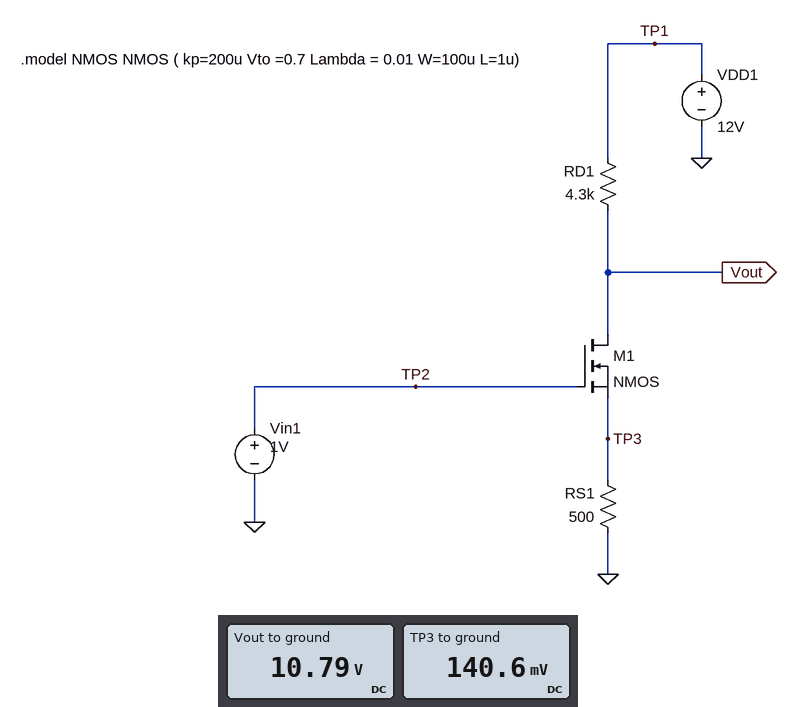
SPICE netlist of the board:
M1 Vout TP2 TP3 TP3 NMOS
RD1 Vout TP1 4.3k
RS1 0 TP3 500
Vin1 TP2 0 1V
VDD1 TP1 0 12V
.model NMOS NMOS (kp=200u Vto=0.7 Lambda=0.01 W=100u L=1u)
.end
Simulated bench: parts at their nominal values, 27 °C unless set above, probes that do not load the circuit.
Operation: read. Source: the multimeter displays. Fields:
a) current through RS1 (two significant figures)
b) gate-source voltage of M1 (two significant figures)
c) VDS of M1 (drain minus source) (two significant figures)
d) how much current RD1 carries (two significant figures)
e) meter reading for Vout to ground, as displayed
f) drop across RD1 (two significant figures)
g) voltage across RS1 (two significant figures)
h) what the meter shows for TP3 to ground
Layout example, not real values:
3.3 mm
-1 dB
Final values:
280 µA
860 mV
11 V
280 µA
10.79 V
1.2 V
140 mV
140.6 mV
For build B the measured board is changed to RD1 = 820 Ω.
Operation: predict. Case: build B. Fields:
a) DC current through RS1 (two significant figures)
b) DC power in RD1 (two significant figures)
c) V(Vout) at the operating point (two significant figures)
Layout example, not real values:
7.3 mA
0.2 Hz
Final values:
280 µA
65 µW
12 V
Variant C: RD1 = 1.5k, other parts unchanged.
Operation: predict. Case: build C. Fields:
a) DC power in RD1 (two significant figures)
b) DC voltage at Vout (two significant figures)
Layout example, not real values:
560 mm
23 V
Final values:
120 µW
12 V
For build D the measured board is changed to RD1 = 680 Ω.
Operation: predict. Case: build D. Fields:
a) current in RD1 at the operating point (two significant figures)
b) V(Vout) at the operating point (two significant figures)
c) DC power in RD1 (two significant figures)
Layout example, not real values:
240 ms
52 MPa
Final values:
280 µA
12 V
54 µW
